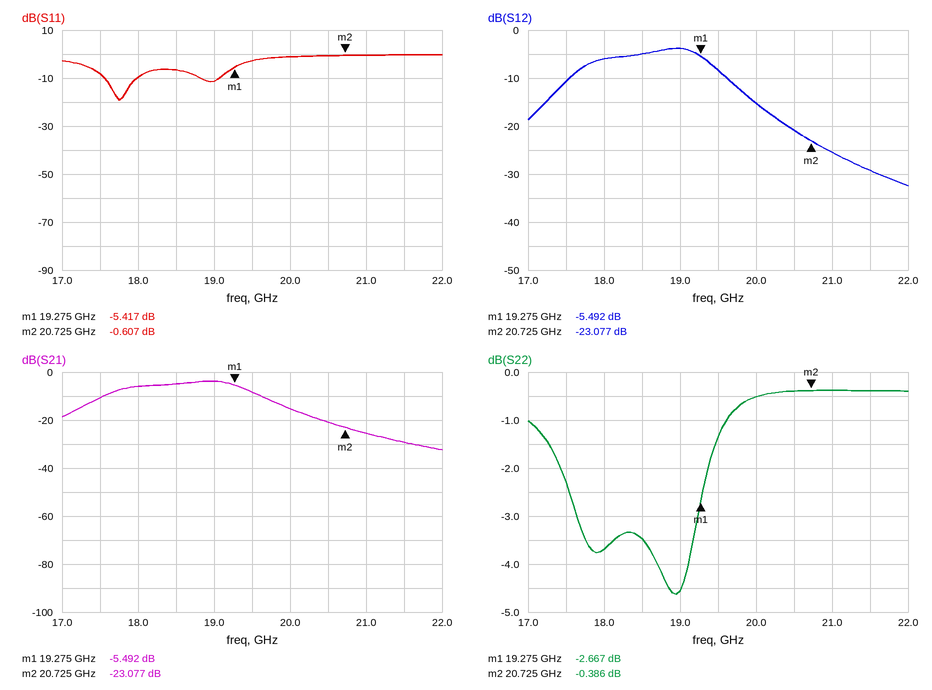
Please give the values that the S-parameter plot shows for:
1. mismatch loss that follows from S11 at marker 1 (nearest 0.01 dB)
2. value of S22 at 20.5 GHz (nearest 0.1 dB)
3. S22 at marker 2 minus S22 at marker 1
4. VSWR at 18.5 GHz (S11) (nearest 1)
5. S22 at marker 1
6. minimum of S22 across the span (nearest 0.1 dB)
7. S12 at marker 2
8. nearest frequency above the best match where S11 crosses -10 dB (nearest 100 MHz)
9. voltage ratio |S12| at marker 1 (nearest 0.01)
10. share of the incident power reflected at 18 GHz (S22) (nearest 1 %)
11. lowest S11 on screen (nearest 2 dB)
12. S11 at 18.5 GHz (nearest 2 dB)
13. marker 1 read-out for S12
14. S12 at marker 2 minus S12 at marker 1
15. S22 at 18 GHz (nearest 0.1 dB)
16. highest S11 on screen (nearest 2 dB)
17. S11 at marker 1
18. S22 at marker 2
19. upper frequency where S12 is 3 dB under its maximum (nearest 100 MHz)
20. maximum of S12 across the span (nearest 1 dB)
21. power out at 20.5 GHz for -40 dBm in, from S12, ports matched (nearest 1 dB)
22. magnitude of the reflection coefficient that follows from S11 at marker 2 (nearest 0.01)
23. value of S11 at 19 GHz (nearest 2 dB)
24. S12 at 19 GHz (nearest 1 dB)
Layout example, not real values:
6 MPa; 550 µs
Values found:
1.47 dB; -0.4 dB; 2.281 dB; 3; -2.667 dB; -4.6 dB; -23.077 dB; 18.0 GHz; 0.53; 43 %; -20 dB; -6 dB; -5.492 dB; -17.585 dB; -3.7 dB; 0 dB; -5.417 dB; -0.386 dB; 19.4 GHz; -4 dB; -61 dBm; 0.93; -12 dB; -4 dB
